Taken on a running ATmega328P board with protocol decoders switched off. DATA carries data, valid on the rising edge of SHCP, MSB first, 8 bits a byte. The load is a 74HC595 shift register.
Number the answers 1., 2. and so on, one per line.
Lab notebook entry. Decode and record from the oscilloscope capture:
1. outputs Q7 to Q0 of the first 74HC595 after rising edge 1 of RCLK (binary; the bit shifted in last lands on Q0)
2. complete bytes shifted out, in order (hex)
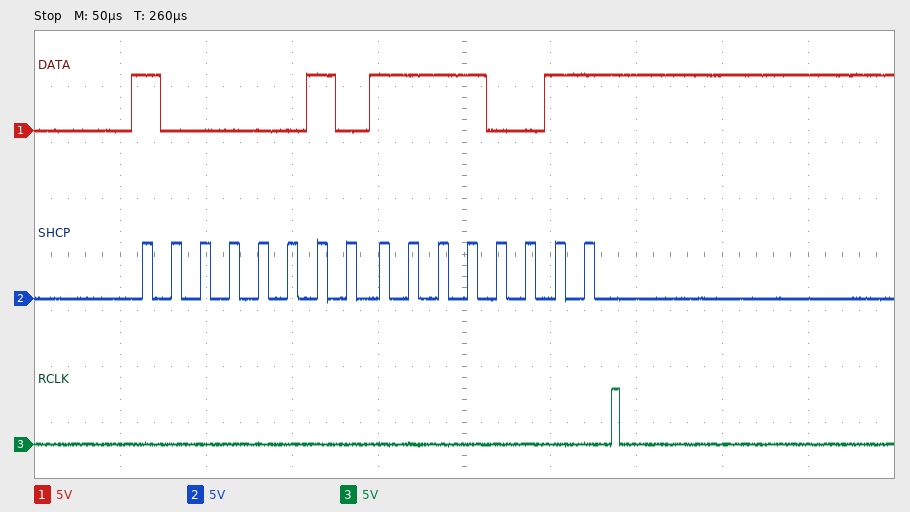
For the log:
1. 11110011
2. 82 F3
